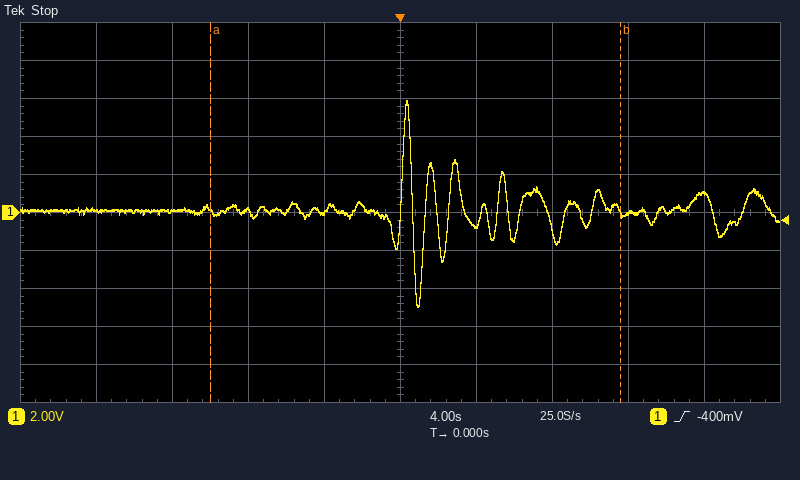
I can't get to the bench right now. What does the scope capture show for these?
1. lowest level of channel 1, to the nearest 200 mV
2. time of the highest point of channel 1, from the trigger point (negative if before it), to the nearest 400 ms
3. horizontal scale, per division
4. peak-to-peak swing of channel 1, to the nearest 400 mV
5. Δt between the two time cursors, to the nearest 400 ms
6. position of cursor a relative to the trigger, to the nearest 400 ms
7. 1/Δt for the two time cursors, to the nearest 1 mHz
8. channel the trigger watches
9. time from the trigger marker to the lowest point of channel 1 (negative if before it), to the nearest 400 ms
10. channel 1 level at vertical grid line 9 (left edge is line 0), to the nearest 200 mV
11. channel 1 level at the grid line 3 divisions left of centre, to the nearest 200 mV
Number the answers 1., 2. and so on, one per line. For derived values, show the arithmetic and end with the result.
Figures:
1. -5.0 V
2. +400 ms
3. 4 s
4. 10.8 V
5. 21.6 s
6. -10.0 s
7. 1 / 21.6 s ≈ 46 mHz
8. channel 1
9. +800 ms
10. 1.0 V
11. 0.0 V
